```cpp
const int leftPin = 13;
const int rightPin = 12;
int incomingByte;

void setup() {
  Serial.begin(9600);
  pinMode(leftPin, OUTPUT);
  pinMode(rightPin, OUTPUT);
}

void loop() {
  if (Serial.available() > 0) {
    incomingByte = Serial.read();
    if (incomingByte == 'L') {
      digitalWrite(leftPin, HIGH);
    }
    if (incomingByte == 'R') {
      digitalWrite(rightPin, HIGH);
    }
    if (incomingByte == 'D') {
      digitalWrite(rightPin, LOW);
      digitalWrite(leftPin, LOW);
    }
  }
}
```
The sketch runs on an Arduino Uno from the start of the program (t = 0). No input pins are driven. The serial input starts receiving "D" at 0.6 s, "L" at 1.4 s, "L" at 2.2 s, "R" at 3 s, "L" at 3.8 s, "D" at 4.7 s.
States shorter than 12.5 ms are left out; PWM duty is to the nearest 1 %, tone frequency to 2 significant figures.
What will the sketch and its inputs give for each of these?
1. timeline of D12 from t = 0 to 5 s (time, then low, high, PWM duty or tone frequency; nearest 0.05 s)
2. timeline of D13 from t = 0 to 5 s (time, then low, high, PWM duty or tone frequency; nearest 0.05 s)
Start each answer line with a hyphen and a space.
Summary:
- 0 s low; 3 s high; 4.7 s low
- 0 s low; 1.4 s high; 4.7 s low
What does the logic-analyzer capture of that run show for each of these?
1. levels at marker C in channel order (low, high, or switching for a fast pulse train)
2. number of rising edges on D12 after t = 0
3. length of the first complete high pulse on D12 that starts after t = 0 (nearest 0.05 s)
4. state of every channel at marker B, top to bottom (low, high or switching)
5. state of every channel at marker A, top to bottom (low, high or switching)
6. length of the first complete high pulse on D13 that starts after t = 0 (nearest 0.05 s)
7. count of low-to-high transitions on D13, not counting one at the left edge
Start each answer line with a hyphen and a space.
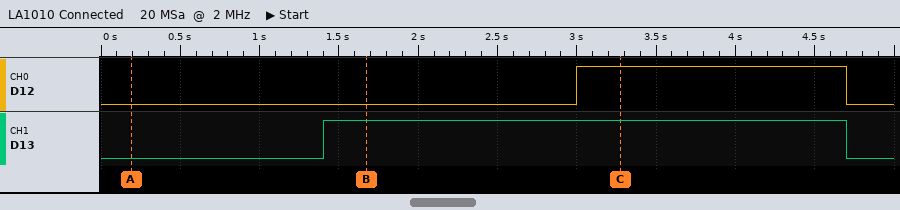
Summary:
- D12 high, D13 high
- 1
- 1.70 s
- D12 low, D13 high
- D12 low, D13 low
- 3.30 s
- 1
